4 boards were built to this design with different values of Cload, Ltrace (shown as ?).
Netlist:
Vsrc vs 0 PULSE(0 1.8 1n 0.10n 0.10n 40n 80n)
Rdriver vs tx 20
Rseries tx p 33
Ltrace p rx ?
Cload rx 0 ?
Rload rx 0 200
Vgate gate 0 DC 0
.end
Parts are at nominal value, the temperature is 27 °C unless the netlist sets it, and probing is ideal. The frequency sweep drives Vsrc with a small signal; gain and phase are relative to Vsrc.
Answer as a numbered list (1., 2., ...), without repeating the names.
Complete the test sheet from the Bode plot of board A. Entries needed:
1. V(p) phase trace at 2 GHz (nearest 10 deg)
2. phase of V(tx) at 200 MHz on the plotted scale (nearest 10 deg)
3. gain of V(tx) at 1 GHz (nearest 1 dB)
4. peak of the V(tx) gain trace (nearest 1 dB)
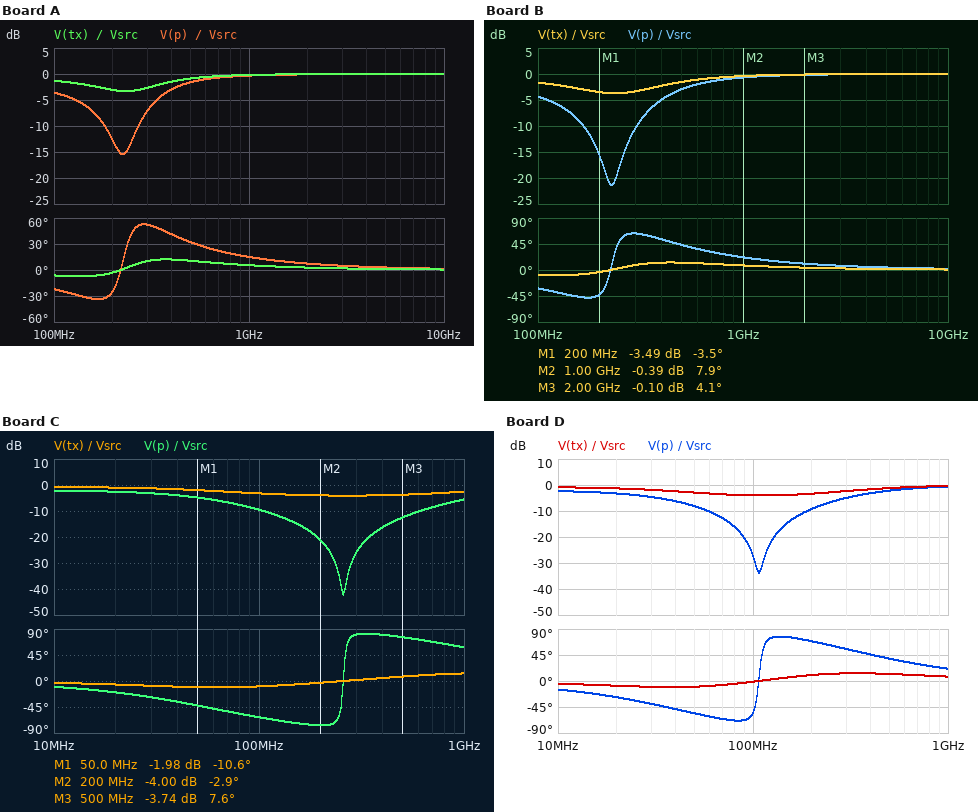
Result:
1. 10 deg
2. 0 deg
3. 0 dB
4. 0 dB
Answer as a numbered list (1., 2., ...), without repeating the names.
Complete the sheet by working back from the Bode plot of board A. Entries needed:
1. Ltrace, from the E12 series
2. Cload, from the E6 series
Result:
1. 33 nH
2. 15 pF
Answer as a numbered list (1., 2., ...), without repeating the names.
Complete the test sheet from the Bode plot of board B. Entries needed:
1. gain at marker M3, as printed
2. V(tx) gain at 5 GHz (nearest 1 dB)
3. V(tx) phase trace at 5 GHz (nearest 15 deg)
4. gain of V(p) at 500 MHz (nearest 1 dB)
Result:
1. -0.10 dB
2. 0 dB
3. 0 deg
4. -3 dB
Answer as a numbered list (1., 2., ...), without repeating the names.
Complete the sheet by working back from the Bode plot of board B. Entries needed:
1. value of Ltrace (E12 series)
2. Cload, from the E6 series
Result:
1. 22 nH
2. 22 pF
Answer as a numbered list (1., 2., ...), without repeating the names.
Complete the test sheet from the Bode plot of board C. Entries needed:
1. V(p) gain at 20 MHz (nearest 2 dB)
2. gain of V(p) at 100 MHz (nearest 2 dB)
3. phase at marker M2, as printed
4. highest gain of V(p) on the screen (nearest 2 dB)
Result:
1. -2 dB
2. -10 dB
3. -2.9 deg
4. -2 dB
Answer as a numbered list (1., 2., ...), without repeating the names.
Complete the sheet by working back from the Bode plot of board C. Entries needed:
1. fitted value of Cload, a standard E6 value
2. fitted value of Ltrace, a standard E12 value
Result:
1. 68 pF
2. 5.6 nH
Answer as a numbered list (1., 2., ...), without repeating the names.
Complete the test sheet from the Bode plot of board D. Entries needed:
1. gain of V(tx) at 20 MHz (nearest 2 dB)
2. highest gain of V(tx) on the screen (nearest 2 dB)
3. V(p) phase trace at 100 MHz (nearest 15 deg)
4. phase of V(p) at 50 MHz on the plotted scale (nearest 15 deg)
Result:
1. -2 dB
2. 0 dB
3. -60 deg
4. -60 deg
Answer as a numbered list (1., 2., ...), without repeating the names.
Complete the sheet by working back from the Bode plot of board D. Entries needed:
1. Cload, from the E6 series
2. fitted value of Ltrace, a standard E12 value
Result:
1. 100 pF
2. 22 nH
